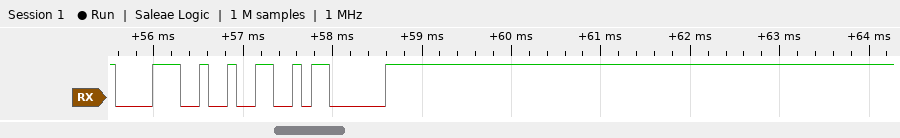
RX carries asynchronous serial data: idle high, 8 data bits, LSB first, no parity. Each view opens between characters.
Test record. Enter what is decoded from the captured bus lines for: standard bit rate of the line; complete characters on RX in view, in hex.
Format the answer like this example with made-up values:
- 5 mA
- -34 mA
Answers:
- 9600 baud
- 38, 32, 03
